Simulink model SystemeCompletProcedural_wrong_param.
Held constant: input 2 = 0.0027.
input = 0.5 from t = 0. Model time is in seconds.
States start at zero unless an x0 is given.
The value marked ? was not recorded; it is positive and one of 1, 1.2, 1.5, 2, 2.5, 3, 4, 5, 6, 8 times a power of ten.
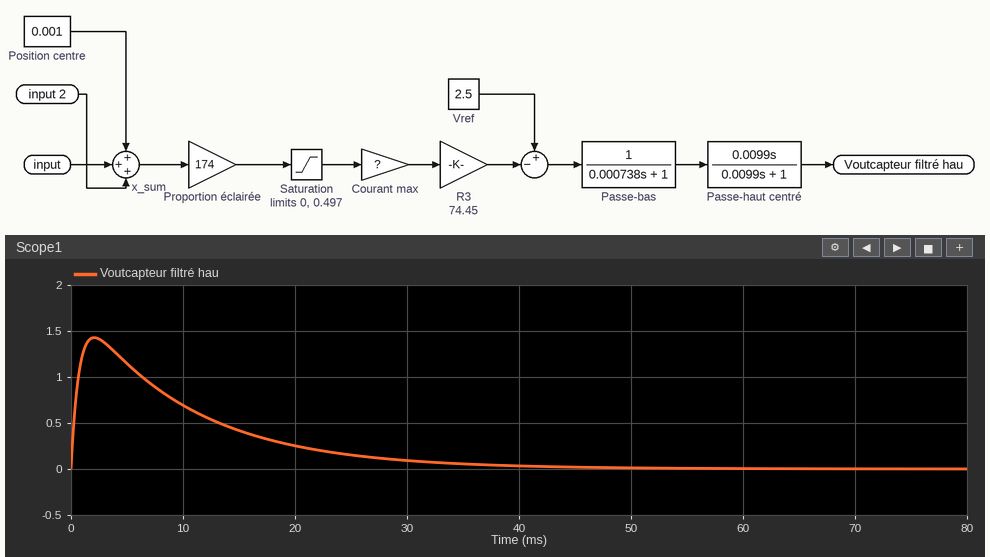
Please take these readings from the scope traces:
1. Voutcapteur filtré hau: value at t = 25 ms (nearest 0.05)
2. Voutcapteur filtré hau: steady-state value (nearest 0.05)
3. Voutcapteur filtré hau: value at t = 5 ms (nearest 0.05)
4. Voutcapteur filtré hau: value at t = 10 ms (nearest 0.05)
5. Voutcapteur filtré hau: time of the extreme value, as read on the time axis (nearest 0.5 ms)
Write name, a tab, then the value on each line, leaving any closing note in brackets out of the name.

Voutcapteur filtré hau: value at t = 25 ms	0.15
Voutcapteur filtré hau: steady-state value	0.00
Voutcapteur filtré hau: value at t = 5 ms	1.15
Voutcapteur filtré hau: value at t = 10 ms	0.70
Voutcapteur filtré hau: time of the extreme value, as read on the time axis	2.0 ms
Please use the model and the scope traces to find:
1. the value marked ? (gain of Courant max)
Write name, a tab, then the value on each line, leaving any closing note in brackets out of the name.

the value marked ?	0.02
